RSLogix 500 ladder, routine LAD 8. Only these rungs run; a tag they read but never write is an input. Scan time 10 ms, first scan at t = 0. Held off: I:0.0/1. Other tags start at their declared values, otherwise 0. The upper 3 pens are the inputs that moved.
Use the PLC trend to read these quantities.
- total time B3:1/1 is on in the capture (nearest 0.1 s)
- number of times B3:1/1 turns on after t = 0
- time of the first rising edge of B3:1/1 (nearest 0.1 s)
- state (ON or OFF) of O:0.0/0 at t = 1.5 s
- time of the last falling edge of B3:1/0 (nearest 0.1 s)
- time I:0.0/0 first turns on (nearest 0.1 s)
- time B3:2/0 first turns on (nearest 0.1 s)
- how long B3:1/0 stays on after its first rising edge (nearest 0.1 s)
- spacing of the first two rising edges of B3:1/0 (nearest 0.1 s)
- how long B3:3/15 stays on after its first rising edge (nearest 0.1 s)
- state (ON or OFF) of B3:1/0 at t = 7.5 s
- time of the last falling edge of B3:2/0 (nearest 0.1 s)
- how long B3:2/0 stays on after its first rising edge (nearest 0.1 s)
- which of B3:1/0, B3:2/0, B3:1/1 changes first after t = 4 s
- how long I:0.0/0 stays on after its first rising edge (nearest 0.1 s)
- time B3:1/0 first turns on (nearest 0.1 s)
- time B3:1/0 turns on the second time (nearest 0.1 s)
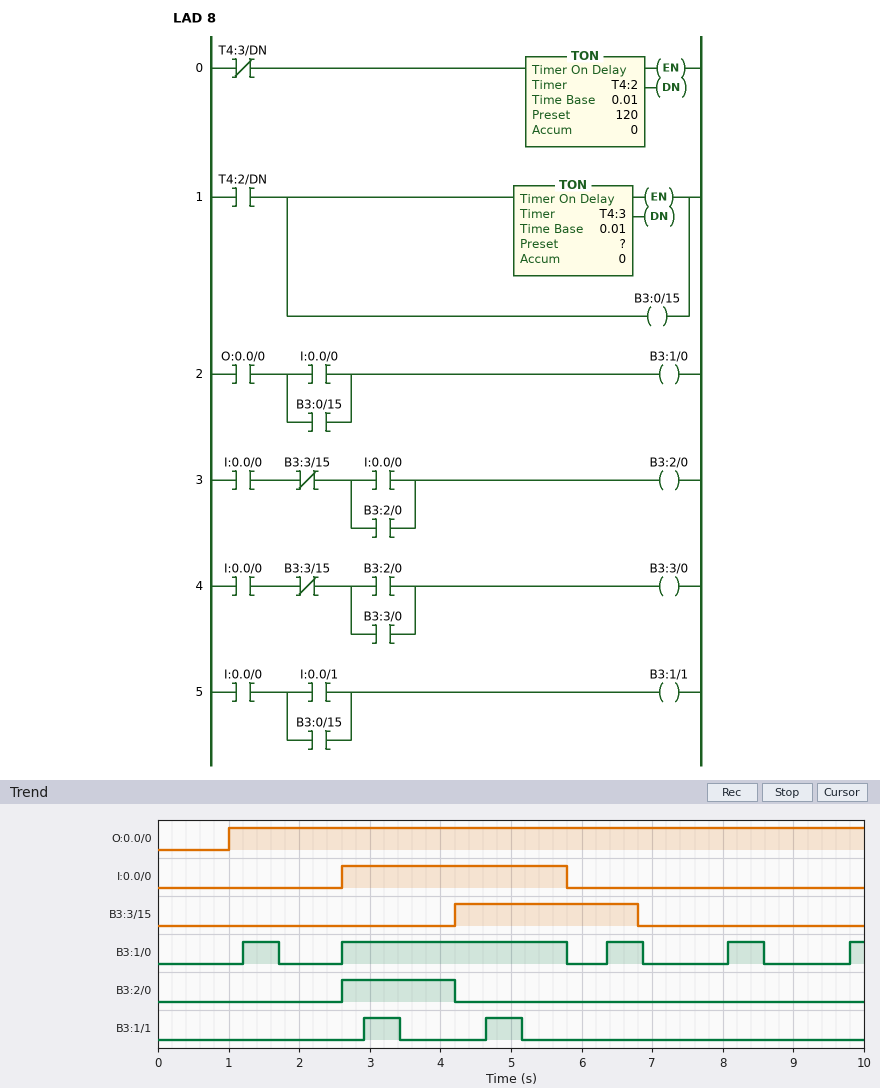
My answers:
1.0 s
2
2.9 s
ON
8.6 s
2.6 s
2.6 s
0.5 s
1.4 s
2.6 s
OFF
4.2 s
1.6 s
B3:2/0
3.2 s
1.2 s
2.6 s
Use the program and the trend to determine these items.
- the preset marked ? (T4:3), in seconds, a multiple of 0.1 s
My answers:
0.5 s
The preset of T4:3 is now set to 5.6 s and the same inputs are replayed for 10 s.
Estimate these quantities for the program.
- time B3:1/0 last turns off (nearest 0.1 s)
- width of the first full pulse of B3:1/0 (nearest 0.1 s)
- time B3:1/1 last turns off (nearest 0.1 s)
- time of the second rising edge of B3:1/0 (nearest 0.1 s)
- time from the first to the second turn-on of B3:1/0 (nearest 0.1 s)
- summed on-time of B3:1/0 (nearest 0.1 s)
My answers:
6.8 s
5.6 s
5.8 s
8.0 s
6.8 s
7.6 s
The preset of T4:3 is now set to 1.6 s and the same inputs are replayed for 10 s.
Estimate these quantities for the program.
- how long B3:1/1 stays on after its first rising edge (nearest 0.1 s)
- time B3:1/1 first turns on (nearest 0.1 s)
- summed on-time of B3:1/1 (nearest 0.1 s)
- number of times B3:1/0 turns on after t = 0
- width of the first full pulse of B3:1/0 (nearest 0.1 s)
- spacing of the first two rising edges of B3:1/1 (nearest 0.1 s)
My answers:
0.2 s
2.6 s
1.8 s
3
4.6 s
1.4 s
